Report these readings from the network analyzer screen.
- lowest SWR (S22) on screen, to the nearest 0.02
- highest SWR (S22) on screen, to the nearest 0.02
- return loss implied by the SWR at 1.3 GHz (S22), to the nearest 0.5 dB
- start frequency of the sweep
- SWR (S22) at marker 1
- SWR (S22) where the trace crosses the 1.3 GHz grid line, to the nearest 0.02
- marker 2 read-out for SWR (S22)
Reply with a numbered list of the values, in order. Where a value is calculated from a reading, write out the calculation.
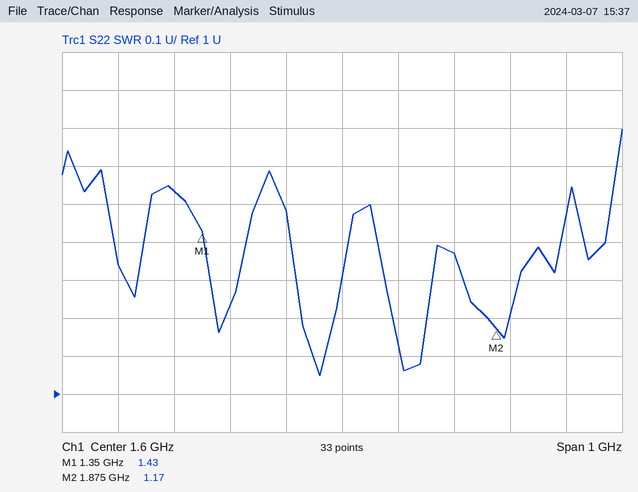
1. 1.04
2. 1.70
3. −20 log10((1.54 − 1)/(1.54 + 1)) ≈ 13.4 dB, so 13.5 dB to the nearest 0.5 dB
4. 1.1 GHz
5. 1.43
6. 1.54
7. 1.17
